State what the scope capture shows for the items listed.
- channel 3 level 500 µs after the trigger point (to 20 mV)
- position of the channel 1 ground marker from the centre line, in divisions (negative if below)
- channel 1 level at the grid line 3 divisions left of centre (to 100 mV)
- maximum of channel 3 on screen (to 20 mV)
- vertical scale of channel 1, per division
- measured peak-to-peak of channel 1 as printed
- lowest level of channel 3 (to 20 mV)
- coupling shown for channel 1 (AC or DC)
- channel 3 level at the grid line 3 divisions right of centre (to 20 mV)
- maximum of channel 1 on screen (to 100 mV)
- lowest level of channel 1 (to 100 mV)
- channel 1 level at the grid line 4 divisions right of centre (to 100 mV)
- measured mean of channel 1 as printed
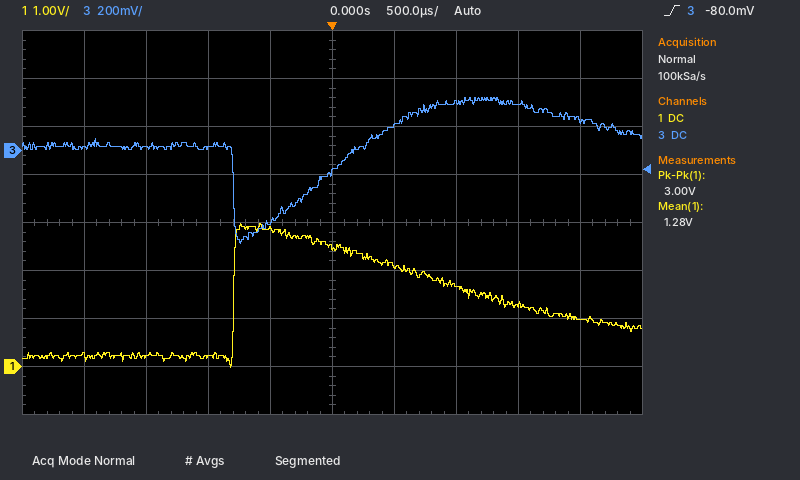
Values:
100 mV
-3.0 div
200 mV
220 mV
1 V
3.00 V
-380 mV
DC
200 mV
3.0 V
0.0 V
1.0 V
1.28 V
